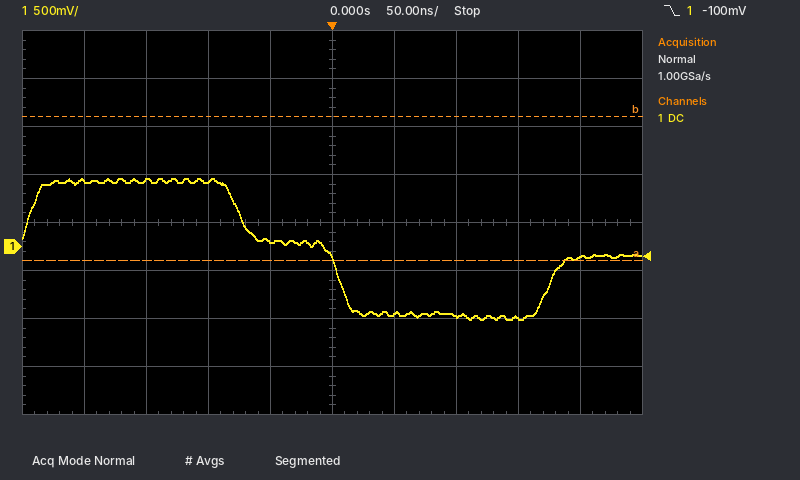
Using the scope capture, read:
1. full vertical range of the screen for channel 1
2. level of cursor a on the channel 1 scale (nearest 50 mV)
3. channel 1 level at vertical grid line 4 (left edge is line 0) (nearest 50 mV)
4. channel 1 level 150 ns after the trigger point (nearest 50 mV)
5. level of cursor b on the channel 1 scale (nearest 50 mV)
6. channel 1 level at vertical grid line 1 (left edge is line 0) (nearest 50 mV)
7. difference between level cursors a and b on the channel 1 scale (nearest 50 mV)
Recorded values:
4 V
-150 mV
50 mV
-750 mV
1.35 V
700 mV
1.50 V
